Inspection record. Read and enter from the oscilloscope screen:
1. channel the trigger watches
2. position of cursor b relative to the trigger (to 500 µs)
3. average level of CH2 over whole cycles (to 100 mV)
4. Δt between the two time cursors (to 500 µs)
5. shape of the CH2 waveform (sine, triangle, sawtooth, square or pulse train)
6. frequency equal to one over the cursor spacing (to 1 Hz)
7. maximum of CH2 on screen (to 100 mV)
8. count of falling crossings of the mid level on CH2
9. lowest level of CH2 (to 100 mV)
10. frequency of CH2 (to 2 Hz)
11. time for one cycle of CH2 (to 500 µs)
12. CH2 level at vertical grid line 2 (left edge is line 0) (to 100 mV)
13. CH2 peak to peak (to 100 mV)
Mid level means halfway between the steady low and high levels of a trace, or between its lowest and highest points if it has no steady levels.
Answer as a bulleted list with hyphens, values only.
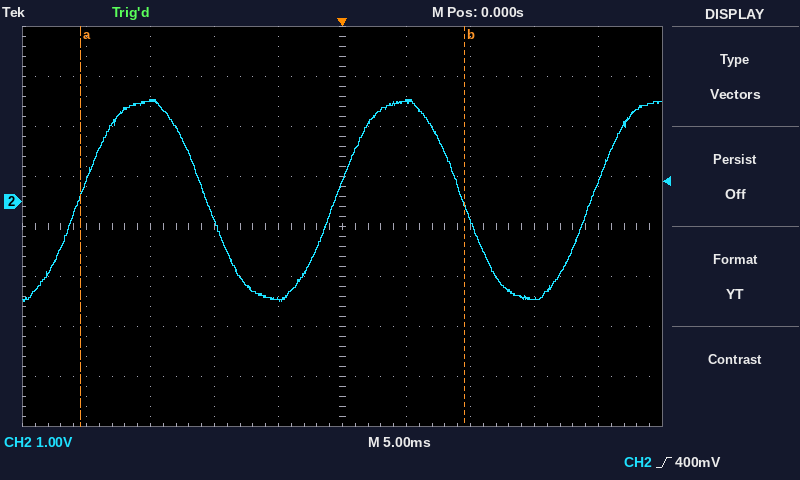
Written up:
- CH2
- +9.5 ms
- 0.0 V
- 30.0 ms
- sine
- 33 Hz
- 2.0 V
- 2
- -2.0 V
- 50 Hz
- 20.0 ms
- 2.0 V
- 4.0 V
